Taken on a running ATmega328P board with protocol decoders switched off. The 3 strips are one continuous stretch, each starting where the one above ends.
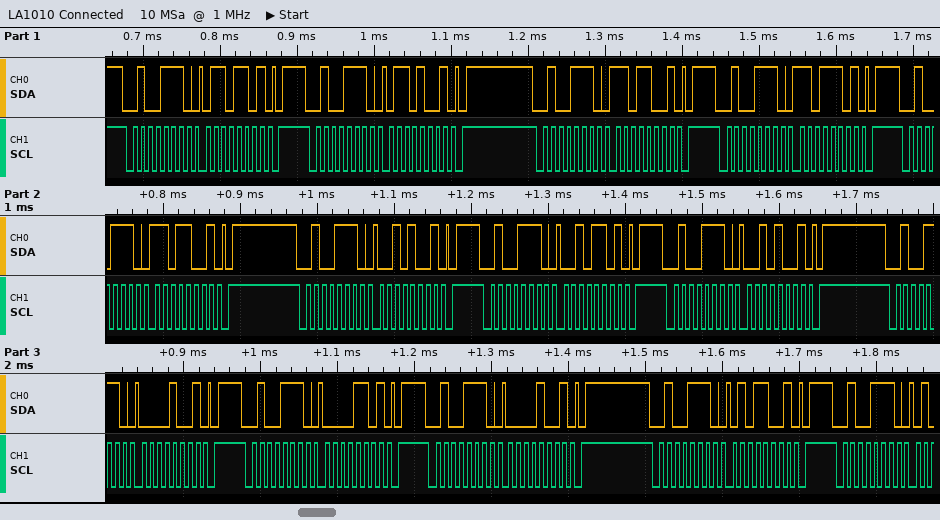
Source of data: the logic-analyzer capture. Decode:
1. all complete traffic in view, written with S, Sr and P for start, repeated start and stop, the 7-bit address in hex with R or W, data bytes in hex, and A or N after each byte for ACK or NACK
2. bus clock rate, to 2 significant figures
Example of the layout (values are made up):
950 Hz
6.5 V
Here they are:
S 27W A 6D A P S 27W A 69 A P S 27W A D9 A P S 27W A DD A P S 27W A D9 A P S 27W A 29 A P S 27W A 2D A P S 27W A 29 A P S 27W A 09 A P S 27W A 0D A P S 27W A 09 A P S 27W A 59 A P S 27W A
100 kHz
